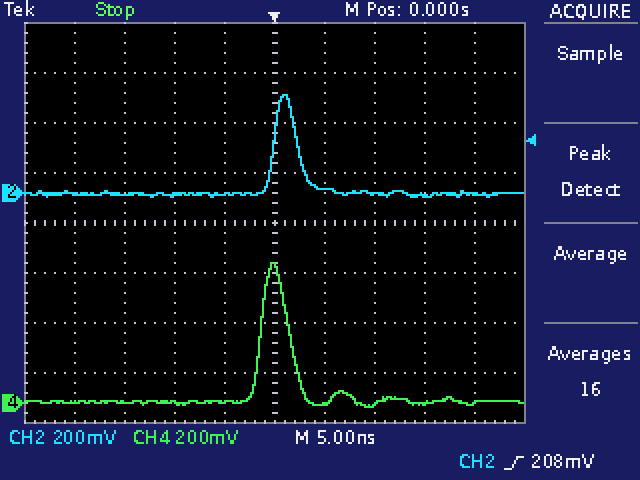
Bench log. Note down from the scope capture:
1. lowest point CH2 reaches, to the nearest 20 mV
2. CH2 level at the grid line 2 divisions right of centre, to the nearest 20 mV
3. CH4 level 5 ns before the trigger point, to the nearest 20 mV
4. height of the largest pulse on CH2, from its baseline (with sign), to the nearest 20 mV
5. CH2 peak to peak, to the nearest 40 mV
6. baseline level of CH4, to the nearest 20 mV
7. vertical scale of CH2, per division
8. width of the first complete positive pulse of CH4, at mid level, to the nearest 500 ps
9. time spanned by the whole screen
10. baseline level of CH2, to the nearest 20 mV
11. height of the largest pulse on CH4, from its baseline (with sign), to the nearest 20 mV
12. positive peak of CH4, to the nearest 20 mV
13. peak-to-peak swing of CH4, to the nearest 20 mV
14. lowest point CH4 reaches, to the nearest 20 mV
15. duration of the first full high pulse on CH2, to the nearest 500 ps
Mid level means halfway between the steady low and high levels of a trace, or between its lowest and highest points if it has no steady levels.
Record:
-20 mV
0 mV
0 mV
+400 mV
400 mV
0 mV
200 mV
3.0 ns
50 ns
0 mV
+560 mV
560 mV
580 mV
-20 mV
2.5 ns
